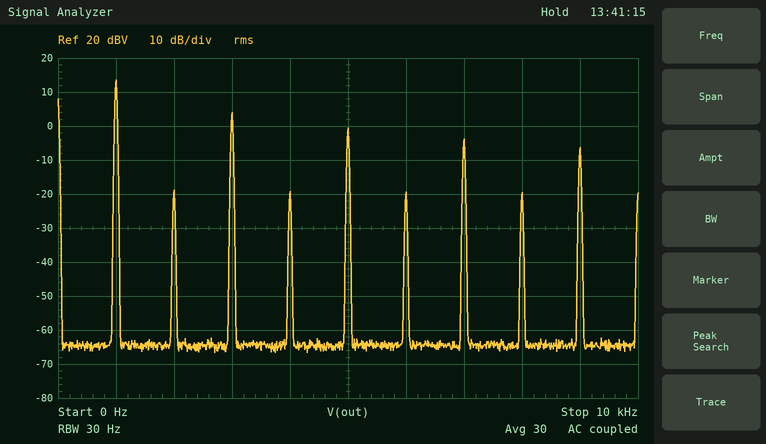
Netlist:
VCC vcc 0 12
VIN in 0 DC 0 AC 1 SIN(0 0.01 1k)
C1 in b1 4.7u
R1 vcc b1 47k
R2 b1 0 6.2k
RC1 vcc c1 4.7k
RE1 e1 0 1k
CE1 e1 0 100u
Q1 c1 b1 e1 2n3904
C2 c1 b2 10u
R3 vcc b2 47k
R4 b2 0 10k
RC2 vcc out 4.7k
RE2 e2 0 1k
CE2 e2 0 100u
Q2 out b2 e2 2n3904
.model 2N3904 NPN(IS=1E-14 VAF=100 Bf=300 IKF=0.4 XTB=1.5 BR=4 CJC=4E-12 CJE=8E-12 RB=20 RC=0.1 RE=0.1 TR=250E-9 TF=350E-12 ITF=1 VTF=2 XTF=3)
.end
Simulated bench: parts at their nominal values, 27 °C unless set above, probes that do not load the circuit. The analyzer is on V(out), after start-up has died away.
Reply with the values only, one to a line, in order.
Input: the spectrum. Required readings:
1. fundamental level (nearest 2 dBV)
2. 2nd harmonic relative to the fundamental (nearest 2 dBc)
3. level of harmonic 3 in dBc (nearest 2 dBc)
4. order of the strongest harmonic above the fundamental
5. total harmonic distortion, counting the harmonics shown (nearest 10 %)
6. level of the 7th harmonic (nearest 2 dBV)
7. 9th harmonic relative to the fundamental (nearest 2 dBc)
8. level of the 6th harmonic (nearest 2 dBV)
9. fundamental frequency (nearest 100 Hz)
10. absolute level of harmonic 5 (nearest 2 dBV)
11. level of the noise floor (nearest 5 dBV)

14 dBV
-32 dBc
-10 dBc
3
40 %
-4 dBV
-20 dBc
-20 dBV
1.0 kHz
0 dBV
-65 dBV
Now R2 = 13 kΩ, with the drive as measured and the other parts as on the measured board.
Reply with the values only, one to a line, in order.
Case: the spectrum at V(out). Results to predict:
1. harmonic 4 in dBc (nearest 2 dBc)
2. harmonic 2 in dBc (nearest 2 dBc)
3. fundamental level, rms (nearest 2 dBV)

-16 dBc
-16 dBc
14 dBV
